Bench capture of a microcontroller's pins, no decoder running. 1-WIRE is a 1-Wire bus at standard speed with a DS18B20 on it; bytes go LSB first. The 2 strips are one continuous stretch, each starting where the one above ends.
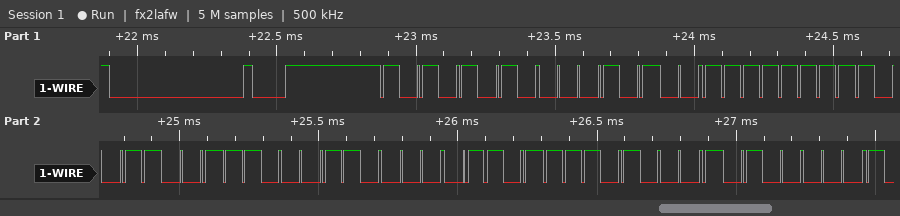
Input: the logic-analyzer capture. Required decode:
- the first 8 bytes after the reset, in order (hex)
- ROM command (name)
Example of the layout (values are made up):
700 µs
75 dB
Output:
55 28 FF 99 63 B0 17 05
Match ROM
